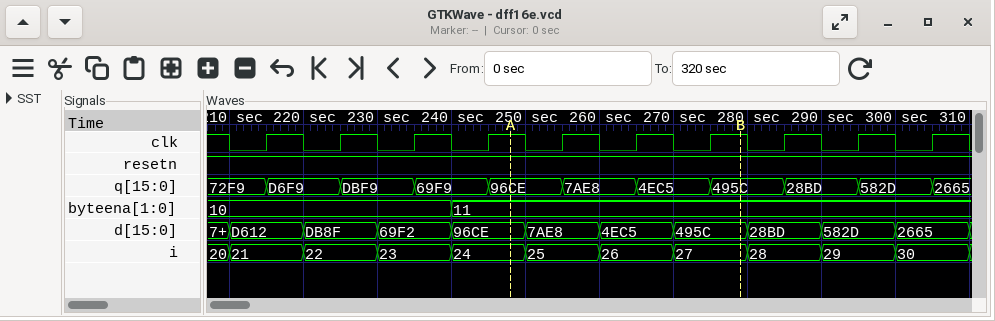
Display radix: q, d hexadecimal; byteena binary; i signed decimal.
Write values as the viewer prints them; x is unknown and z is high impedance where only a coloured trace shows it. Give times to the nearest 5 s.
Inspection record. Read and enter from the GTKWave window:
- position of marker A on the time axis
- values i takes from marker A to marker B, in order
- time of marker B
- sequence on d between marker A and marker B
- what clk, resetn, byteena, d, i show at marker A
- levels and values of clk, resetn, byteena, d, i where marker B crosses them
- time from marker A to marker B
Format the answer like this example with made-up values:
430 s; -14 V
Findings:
250 s; 24, 25, 26, 27; 280 s; 96CE, 7AE8, 4EC5, 495C; clk=1, resetn=1, byteena=11, d=96CE, i=24; clk=1, resetn=1, byteena=11, d=495C, i=27; 30 s
